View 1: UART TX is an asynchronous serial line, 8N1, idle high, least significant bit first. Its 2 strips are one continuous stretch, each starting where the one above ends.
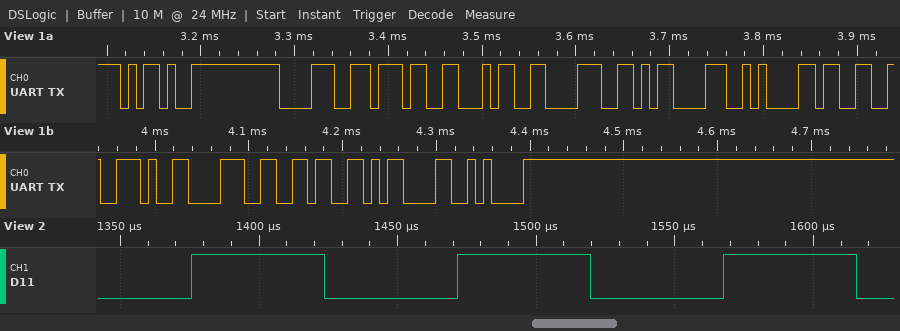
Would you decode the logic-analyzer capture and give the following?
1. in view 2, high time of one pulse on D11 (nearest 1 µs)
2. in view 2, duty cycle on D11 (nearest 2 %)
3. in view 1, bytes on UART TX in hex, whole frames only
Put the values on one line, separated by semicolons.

48 µs; 50 %; 2D 38 37 34 38 0D 0A 33 2E 38 36 0D 0A
